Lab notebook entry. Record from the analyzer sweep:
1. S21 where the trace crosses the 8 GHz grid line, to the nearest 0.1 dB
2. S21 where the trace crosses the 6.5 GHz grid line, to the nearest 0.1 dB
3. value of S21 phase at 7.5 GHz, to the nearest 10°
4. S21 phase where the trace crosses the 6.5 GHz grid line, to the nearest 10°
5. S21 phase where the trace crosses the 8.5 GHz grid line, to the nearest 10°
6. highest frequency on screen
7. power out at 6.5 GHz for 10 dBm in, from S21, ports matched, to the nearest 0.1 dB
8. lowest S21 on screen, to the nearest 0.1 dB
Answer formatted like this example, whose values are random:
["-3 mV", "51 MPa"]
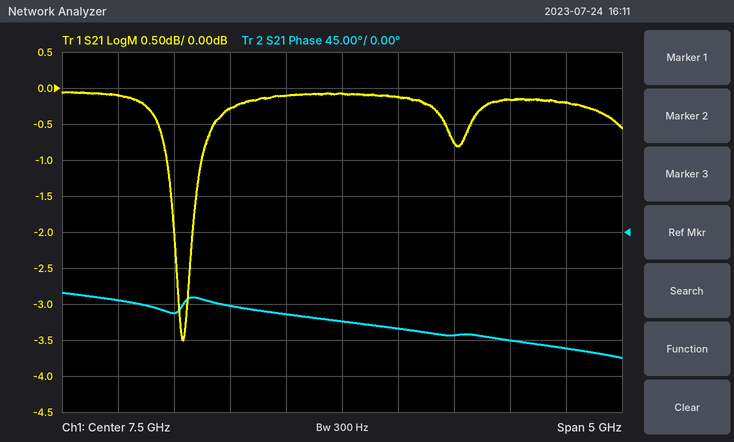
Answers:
["-0.1 dB", "-0.3 dB", "-110°", "-90°", "-130°", "10 GHz", "9.7 dBm", "-3.5 dB"]
